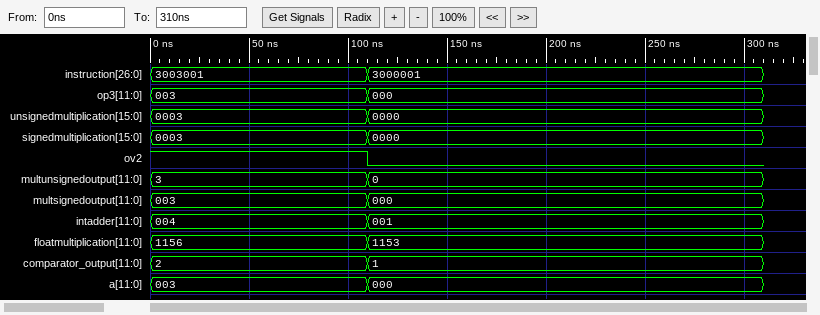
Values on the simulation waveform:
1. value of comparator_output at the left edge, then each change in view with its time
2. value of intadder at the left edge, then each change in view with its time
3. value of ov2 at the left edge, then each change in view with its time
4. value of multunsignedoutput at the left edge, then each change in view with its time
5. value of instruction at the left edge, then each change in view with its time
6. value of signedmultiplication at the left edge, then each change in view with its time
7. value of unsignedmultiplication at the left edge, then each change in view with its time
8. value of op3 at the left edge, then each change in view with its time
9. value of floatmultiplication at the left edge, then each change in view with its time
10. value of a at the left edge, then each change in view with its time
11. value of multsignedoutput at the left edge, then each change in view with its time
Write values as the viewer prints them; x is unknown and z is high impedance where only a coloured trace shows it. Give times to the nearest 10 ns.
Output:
2, 1 at 110 ns
004, 001 at 110 ns
1, 0 at 110 ns
3, 0 at 110 ns
3003001, 3000001 at 110 ns
0003, 0000 at 110 ns
0003, 0000 at 110 ns
003, 000 at 110 ns
1156, 1153 at 110 ns
003, 000 at 110 ns
003, 000 at 110 ns
